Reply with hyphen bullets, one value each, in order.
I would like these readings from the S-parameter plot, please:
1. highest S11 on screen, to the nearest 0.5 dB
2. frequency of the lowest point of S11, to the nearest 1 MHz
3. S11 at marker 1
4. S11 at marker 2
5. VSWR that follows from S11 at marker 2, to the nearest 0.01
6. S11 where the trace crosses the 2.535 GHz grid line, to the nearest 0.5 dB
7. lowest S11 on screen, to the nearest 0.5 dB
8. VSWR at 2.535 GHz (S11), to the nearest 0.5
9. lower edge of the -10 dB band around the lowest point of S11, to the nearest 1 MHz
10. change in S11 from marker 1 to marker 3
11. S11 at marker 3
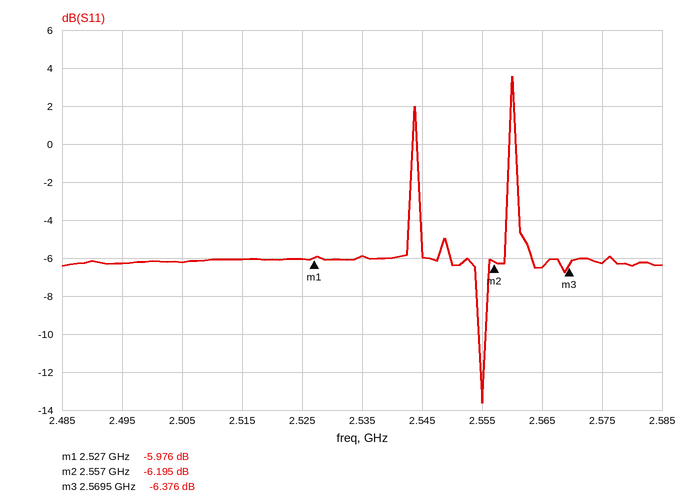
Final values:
- 3.5 dB
- 2.555 GHz
- -5.976 dB
- -6.195 dB
- 2.92
- -6.0 dB
- -13.5 dB
- 3.0
- 2.554 GHz
- -0.400 dB
- -6.376 dB
